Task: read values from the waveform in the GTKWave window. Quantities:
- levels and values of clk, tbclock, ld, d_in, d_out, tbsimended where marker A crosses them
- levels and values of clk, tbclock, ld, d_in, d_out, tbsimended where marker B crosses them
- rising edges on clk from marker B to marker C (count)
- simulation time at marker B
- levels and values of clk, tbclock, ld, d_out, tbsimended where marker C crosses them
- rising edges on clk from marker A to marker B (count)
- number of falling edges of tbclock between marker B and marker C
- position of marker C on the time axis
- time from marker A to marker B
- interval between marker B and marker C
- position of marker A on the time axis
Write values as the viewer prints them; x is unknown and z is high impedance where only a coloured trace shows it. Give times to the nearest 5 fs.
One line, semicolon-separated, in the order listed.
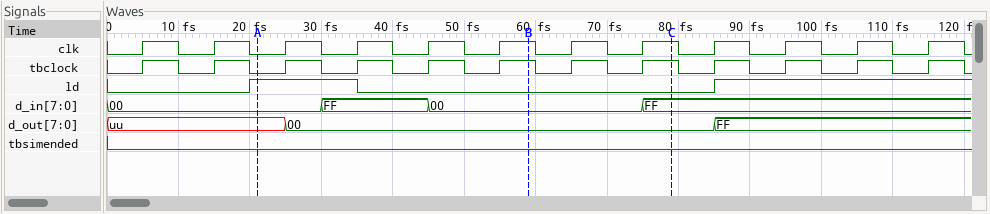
clk=0, tbclock=0, ld=1, d_in=00, d_out=uu, tbsimended=0; clk=1, tbclock=1, ld=0, d_in=00, d_out=00, tbsimended=0; 2; 60 fs; clk=1, tbclock=1, ld=0, d_out=00, tbsimended=0; 4; 2; 80 fs; 40 fs; 20 fs; 20 fs
